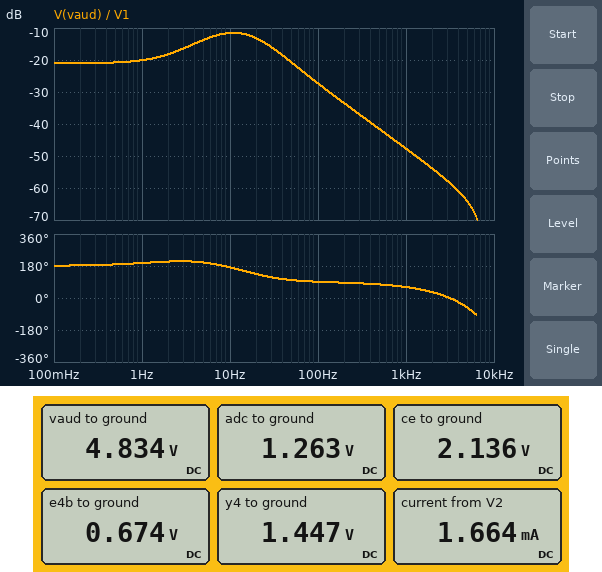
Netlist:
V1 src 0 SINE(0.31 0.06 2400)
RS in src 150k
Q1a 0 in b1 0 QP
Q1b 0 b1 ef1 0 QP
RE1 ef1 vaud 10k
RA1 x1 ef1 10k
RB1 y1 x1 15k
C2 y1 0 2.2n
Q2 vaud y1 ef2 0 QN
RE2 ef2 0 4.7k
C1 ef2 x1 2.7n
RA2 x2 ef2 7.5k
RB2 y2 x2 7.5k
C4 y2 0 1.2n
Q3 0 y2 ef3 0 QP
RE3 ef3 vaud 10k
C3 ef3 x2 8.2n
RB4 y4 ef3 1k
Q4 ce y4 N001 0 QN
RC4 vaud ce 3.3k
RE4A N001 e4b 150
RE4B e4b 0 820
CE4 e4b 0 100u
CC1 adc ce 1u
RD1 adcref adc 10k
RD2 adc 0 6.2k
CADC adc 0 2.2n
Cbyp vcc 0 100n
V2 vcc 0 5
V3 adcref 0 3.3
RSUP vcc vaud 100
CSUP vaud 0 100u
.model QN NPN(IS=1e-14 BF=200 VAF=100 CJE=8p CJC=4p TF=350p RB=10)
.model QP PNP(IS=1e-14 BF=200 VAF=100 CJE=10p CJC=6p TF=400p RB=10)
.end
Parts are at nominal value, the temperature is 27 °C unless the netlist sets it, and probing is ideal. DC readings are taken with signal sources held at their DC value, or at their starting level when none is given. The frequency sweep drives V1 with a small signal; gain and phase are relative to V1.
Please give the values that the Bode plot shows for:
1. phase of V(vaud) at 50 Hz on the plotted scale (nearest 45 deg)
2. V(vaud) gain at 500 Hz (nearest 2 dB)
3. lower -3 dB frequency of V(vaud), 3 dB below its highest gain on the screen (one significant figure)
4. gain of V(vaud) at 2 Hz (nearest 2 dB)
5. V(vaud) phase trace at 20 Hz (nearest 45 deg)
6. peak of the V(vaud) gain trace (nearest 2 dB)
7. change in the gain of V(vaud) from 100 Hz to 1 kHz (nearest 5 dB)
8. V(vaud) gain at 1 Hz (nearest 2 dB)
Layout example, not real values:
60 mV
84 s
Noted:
90 deg
-42 dB
4 Hz
-18 dB
135 deg
-12 dB
-20 dB
-20 dB
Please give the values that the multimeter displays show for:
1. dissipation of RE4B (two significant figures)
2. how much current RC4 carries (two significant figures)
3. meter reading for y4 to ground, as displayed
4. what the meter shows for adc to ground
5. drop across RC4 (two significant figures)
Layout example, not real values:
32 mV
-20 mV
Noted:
550 µW
820 µA
1.447 V
1.263 V
2.7 V
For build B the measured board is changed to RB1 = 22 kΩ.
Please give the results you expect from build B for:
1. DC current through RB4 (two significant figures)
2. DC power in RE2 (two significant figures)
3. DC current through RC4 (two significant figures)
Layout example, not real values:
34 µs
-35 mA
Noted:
4.0 µA
130 µW
810 µA
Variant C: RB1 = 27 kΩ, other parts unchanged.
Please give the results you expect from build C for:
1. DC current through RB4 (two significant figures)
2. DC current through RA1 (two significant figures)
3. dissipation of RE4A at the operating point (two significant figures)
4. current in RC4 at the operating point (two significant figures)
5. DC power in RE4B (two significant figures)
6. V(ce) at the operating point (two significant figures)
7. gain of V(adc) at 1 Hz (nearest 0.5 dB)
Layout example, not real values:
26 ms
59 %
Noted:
4.0 µA
800 nA
99 µW
810 µA
540 µW
2.2 V
-22.0 dB
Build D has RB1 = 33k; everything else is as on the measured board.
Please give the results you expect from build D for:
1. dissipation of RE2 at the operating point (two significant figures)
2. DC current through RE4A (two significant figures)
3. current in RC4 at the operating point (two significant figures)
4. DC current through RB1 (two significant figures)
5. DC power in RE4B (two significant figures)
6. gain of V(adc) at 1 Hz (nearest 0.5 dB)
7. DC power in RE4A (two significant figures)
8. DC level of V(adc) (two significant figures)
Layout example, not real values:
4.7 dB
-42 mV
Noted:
130 µW
810 µA
800 µA
800 nA
540 µW
-22.0 dB
98 µW
1.3 V
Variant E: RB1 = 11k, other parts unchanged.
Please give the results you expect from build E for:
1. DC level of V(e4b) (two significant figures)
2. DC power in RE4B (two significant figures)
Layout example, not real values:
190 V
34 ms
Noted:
680 mV
560 µW
